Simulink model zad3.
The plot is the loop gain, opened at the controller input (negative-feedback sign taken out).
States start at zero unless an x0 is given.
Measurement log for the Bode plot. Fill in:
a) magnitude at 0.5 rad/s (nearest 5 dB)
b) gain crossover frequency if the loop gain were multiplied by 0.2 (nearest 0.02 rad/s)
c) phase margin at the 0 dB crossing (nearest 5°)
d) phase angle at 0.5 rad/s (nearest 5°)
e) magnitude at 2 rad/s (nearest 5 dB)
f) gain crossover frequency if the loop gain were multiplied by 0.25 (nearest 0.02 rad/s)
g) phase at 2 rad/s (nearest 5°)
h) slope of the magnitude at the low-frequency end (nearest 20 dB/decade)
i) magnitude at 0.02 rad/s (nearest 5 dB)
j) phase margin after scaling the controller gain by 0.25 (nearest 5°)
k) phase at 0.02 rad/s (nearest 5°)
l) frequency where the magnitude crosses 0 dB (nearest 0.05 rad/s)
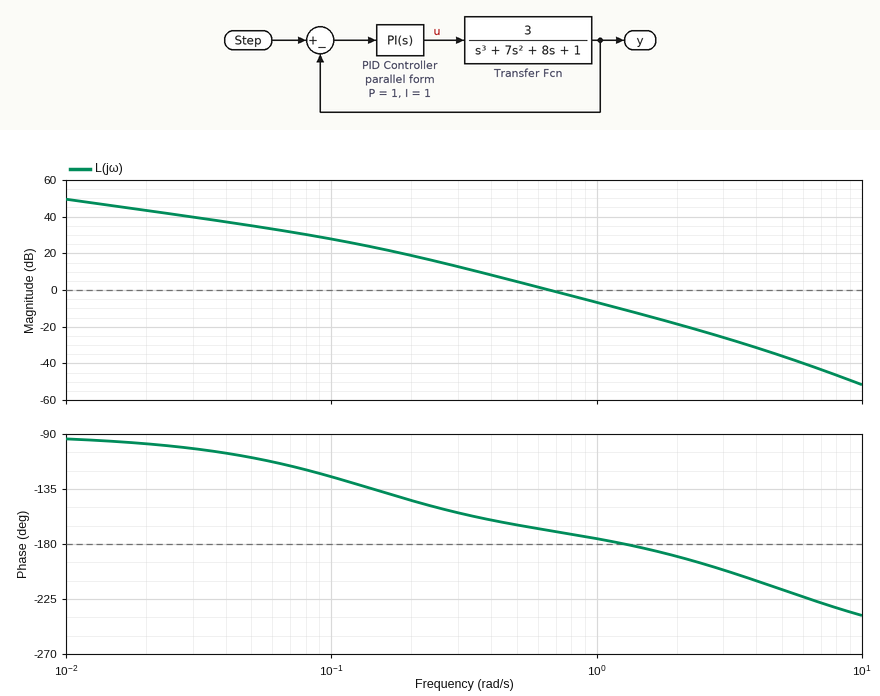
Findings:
5 dB
0.28 rad/s
10°
-165°
-20 dB
0.32 rad/s
-190°
-20 dB/decade
45 dB
25°
-100°
0.65 rad/s
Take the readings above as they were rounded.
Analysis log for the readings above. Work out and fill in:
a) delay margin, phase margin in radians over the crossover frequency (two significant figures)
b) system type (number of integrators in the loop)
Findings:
0.27 s
1
